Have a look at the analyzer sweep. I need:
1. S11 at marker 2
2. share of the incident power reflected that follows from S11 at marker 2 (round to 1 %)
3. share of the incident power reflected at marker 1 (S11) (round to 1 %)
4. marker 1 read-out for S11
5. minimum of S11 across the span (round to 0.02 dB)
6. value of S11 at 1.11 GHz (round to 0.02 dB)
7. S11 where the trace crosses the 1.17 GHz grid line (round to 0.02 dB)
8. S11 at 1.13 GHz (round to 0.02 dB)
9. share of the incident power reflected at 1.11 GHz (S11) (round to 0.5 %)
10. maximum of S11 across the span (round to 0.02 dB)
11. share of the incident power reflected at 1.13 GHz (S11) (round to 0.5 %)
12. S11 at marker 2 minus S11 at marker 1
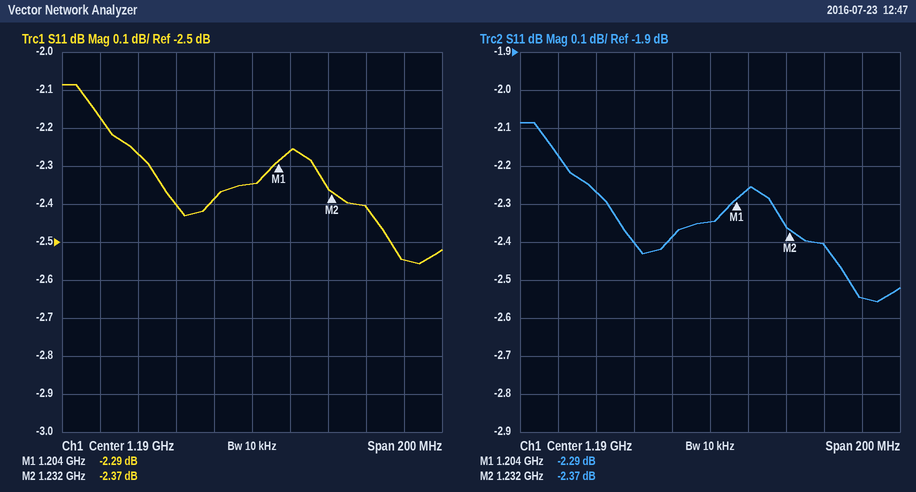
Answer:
-2.37 dB
58 %
59 %
-2.29 dB
-2.56 dB
-2.18 dB
-2.38 dB
-2.26 dB
60.5 %
-2.08 dB
59.5 %
-0.08 dB
